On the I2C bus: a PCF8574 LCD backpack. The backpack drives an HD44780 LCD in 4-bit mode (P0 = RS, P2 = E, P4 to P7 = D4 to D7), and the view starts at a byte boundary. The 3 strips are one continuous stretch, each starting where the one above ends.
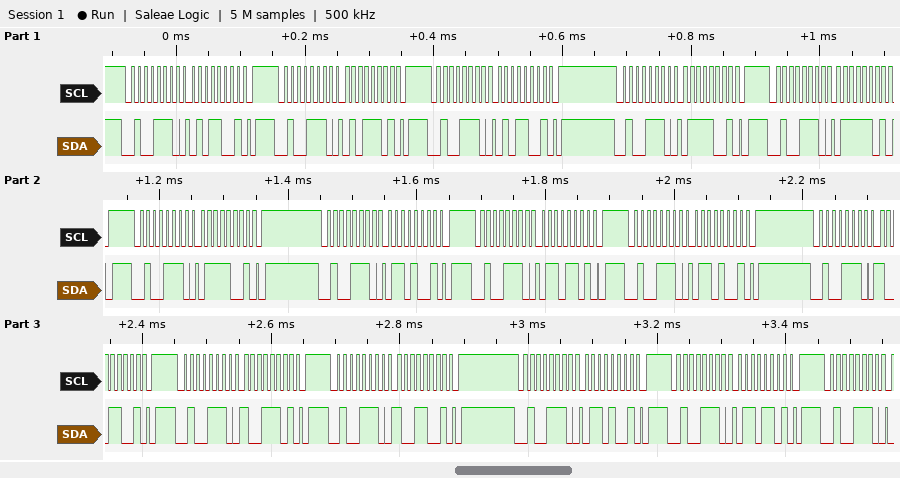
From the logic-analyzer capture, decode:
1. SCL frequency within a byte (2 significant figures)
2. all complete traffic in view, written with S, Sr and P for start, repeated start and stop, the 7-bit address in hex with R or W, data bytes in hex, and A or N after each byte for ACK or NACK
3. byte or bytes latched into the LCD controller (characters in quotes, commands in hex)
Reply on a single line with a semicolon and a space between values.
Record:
100 kHz; S 27W A 59 A P S 27W A 5D A P S 27W A 59 A P S 27W A 79 A P S 27W A 7D A P S 27W A 79 A P S 27W A 69 A P S 27W A 6D A P S 27W A 69 A P S 27W A 99 A P S 27W A 9D A P S 27W A 99 A P S 27W A 69 A P S 27W A 6D A P S 27W A; 'W' 'i'
